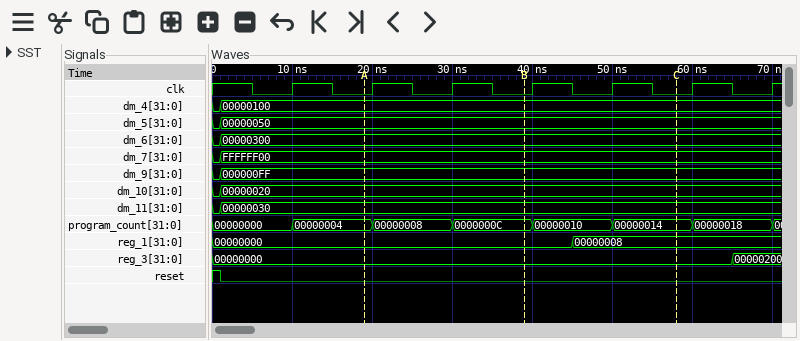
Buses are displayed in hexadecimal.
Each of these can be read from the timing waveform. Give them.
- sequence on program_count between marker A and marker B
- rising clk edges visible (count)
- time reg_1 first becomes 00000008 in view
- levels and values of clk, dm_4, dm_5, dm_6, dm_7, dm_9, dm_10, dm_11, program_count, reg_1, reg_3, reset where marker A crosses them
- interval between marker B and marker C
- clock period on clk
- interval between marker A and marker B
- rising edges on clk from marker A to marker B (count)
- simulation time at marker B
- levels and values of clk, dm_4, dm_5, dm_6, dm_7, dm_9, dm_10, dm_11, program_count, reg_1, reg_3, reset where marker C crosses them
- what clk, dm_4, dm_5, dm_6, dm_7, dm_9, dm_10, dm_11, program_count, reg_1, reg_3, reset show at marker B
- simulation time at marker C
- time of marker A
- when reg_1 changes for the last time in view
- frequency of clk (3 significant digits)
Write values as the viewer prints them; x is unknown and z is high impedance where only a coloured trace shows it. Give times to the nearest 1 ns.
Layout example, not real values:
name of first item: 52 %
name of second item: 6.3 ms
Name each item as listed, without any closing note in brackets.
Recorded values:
sequence on program_count between marker A and marker B: 00000004, 00000008, 0000000C
rising clk edges visible: 7
time reg_1 first becomes 00000008 in view: 45 ns
levels and values of clk, dm_4, dm_5, dm_6, dm_7, dm_9, dm_10, dm_11, program_count, reg_1, reg_3, reset where marker A crosses them: clk=0, dm_4=00000100, dm_5=00000050, dm_6=00000300, dm_7=FFFFFF00, dm_9=000000FF, dm_10=00000020, dm_11=00000030, program_count=00000004, reg_1=00000000, reg_3=00000000, reset=0
interval between marker B and marker C: 19 ns
clock period on clk: 10 ns
interval between marker A and marker B: 20 ns
rising edges on clk from marker A to marker B: 2
simulation time at marker B: 39 ns
levels and values of clk, dm_4, dm_5, dm_6, dm_7, dm_9, dm_10, dm_11, program_count, reg_1, reg_3, reset where marker C crosses them: clk=0, dm_4=00000100, dm_5=00000050, dm_6=00000300, dm_7=FFFFFF00, dm_9=000000FF, dm_10=00000020, dm_11=00000030, program_count=00000014, reg_1=00000008, reg_3=00000000, reset=0
what clk, dm_4, dm_5, dm_6, dm_7, dm_9, dm_10, dm_11, program_count, reg_1, reg_3, reset show at marker B: clk=0, dm_4=00000100, dm_5=00000050, dm_6=00000300, dm_7=FFFFFF00, dm_9=000000FF, dm_10=00000020, dm_11=00000030, program_count=0000000C, reg_1=00000000, reg_3=00000000, reset=0
simulation time at marker C: 58 ns
time of marker A: 19 ns
when reg_1 changes for the last time in view: 45 ns
frequency of clk: 100 MHz
